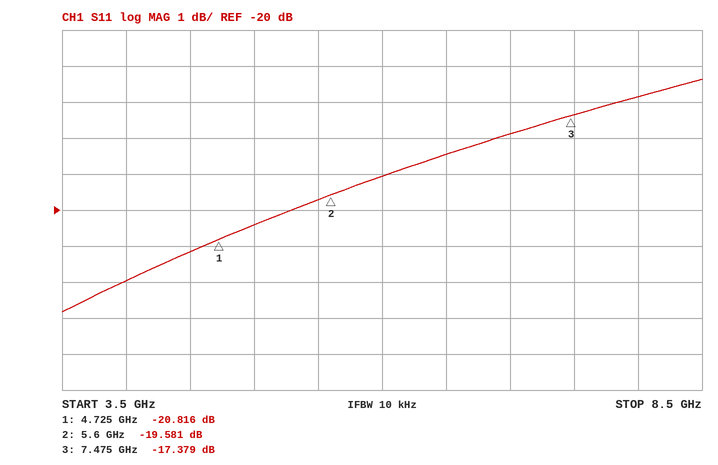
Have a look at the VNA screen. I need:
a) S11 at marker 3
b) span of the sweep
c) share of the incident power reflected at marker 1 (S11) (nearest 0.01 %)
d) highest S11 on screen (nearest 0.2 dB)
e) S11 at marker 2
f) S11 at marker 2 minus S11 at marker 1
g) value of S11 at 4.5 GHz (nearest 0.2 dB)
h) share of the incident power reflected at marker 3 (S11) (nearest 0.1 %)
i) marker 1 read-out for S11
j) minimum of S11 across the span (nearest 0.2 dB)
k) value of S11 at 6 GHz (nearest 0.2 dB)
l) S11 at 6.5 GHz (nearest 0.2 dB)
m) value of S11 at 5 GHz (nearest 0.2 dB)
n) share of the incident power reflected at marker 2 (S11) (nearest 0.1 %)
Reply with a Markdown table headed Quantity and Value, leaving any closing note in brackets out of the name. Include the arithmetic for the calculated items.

| Quantity | Value |
|---|---|
| S11 at marker 3 | -17.379 dB |
| span of the sweep | 5 GHz |
| share of the incident power reflected at marker 1 (S11) | 10^(-20.816/10) ≈ 0.83 % |
| highest S11 on screen | -16.4 dB |
| S11 at marker 2 | -19.581 dB |
| S11 at marker 2 minus S11 at marker 1 | -19.581 − (-20.816) = 1.235 dB |
| value of S11 at 4.5 GHz | -21.2 dB |
| share of the incident power reflected at marker 3 (S11) | 10^(-17.379/10) ≈ 1.8 % |
| marker 1 read-out for S11 | -20.816 dB |
| minimum of S11 across the span | -22.8 dB |
| value of S11 at 6 GHz | -19.0 dB |
| S11 at 6.5 GHz | -18.4 dB |
| value of S11 at 5 GHz | -20.4 dB |
| share of the incident power reflected at marker 2 (S11) | 10^(-19.581/10) ≈ 1.1 % |
